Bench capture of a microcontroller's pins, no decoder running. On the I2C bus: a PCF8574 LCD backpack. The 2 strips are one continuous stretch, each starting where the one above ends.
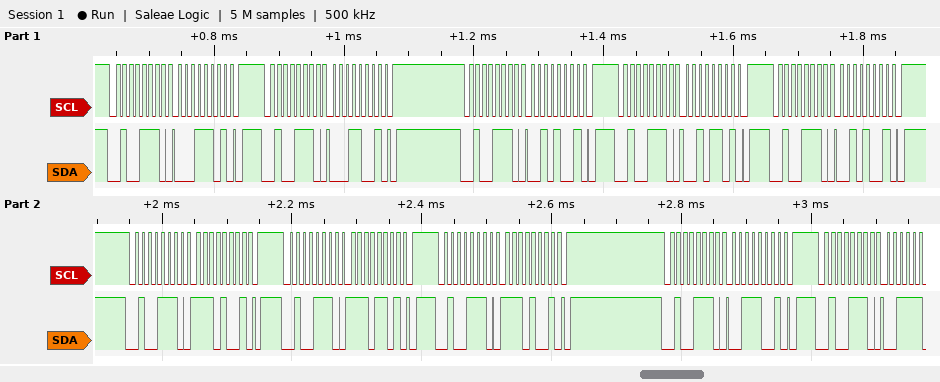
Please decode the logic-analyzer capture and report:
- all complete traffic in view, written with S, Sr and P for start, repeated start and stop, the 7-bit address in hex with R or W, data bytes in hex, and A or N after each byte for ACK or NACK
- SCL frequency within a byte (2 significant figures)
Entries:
S 27W A 1D A P S 27W A 19 A P S 27W A 29 A P S 27W A 2D A P S 27W A 29 A P S 27W A E9 A P S 27W A ED A P S 27W A E9 A P S 27W A 39 A P S 27W A
100 kHz
